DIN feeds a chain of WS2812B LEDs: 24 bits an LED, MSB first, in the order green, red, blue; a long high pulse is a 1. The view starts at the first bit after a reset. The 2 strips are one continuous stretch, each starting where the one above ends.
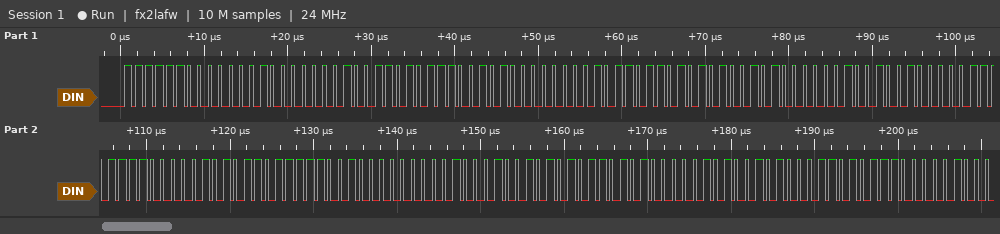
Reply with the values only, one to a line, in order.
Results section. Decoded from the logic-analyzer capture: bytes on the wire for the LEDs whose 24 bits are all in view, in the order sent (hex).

FC 04 04 D7 28 05 B5 4A 04 90 6F 05 6F 90 04 4A B5 05 28 D7 04
